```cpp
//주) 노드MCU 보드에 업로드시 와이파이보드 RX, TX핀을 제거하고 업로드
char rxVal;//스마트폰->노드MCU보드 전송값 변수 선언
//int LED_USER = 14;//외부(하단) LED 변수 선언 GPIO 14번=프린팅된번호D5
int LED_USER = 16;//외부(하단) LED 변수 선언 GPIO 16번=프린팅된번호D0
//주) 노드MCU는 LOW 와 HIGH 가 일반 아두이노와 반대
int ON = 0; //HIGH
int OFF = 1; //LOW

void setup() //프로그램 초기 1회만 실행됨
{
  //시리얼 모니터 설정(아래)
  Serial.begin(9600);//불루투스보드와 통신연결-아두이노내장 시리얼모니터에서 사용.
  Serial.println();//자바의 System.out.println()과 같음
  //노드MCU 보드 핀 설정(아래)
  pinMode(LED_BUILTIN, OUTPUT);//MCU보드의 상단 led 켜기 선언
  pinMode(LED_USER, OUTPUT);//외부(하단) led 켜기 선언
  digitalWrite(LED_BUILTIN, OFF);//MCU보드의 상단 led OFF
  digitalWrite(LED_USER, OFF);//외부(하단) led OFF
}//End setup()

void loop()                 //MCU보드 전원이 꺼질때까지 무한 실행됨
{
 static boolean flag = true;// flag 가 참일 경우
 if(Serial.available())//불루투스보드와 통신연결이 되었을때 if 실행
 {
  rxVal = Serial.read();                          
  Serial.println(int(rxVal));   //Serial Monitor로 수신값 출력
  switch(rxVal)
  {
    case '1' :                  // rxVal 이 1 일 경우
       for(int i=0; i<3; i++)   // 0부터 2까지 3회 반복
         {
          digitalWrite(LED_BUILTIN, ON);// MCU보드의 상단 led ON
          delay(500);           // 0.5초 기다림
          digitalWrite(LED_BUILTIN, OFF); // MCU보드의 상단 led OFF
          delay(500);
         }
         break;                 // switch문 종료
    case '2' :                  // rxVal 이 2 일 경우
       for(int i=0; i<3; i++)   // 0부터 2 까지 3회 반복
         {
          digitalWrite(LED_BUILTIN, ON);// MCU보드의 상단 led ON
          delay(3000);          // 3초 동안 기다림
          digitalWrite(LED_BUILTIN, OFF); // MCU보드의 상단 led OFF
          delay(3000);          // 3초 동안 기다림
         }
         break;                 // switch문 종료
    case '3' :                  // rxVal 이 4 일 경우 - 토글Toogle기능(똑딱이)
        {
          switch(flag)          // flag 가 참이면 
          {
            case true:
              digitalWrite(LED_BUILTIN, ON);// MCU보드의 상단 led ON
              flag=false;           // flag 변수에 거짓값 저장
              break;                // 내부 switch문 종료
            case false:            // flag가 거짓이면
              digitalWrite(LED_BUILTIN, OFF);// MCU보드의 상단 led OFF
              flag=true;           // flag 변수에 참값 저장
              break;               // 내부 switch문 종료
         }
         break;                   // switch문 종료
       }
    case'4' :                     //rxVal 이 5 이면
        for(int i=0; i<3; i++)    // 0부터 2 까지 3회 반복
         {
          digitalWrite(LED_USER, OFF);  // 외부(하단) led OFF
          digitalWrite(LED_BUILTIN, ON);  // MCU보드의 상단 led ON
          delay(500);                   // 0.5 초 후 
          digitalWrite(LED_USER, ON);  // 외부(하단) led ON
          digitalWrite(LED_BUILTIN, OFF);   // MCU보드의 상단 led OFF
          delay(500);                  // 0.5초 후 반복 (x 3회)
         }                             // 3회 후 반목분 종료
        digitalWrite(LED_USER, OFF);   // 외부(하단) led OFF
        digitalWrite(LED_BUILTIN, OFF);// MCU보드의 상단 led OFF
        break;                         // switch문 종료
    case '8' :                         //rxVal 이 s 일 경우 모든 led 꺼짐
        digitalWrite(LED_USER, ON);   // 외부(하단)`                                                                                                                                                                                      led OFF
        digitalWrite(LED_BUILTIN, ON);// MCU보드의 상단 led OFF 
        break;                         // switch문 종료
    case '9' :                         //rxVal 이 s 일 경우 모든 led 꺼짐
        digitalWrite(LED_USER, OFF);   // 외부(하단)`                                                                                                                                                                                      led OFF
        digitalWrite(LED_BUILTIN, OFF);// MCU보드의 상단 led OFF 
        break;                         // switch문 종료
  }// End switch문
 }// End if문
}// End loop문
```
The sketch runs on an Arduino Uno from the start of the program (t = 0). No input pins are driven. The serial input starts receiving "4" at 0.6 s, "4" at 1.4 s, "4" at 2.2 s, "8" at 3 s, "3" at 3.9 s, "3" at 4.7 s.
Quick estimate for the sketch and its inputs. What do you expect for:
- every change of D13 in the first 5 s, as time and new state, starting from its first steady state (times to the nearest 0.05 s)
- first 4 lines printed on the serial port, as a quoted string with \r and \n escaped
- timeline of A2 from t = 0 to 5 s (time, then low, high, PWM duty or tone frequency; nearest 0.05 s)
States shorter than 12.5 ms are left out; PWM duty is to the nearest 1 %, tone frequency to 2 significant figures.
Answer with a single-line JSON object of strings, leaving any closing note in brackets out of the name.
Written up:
{"every change of D13 in the first 5 s, as time and new state, starting from its first steady state": "0 s high; 0.6 s low; 1.1 s high; 1.6 s low; 2.1 s high; 2.6 s low; 3.1 s high; 3.6 s low; 4.1 s high; 4.6 s low", "first 4 lines printed on the serial port, as a quoted string with \\r and \\n escaped": "\"\\r\\n52\\r\\n52\\r\\n52\\r\\n\"", "timeline of A2 from t = 0 to 5 s": "0 s high; 1.1 s low; 1.6 s high; 2.1 s low; 2.6 s high; 3.1 s low; 3.6 s high; 4.1 s low; 4.6 s high"}
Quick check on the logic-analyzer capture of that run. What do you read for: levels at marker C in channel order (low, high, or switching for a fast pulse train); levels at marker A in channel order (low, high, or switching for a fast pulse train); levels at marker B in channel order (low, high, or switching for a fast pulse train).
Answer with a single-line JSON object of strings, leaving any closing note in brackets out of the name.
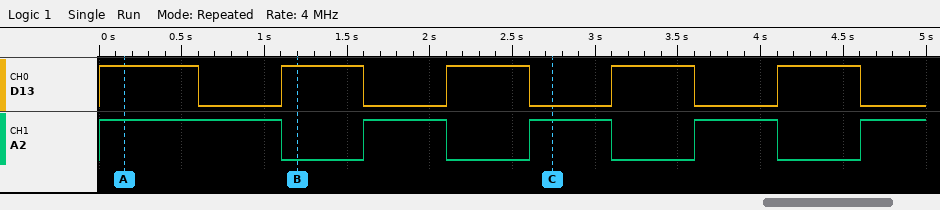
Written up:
{"levels at marker C in channel order": "D13 low, A2 high", "levels at marker A in channel order": "D13 high, A2 high", "levels at marker B in channel order": "D13 high, A2 low"}
